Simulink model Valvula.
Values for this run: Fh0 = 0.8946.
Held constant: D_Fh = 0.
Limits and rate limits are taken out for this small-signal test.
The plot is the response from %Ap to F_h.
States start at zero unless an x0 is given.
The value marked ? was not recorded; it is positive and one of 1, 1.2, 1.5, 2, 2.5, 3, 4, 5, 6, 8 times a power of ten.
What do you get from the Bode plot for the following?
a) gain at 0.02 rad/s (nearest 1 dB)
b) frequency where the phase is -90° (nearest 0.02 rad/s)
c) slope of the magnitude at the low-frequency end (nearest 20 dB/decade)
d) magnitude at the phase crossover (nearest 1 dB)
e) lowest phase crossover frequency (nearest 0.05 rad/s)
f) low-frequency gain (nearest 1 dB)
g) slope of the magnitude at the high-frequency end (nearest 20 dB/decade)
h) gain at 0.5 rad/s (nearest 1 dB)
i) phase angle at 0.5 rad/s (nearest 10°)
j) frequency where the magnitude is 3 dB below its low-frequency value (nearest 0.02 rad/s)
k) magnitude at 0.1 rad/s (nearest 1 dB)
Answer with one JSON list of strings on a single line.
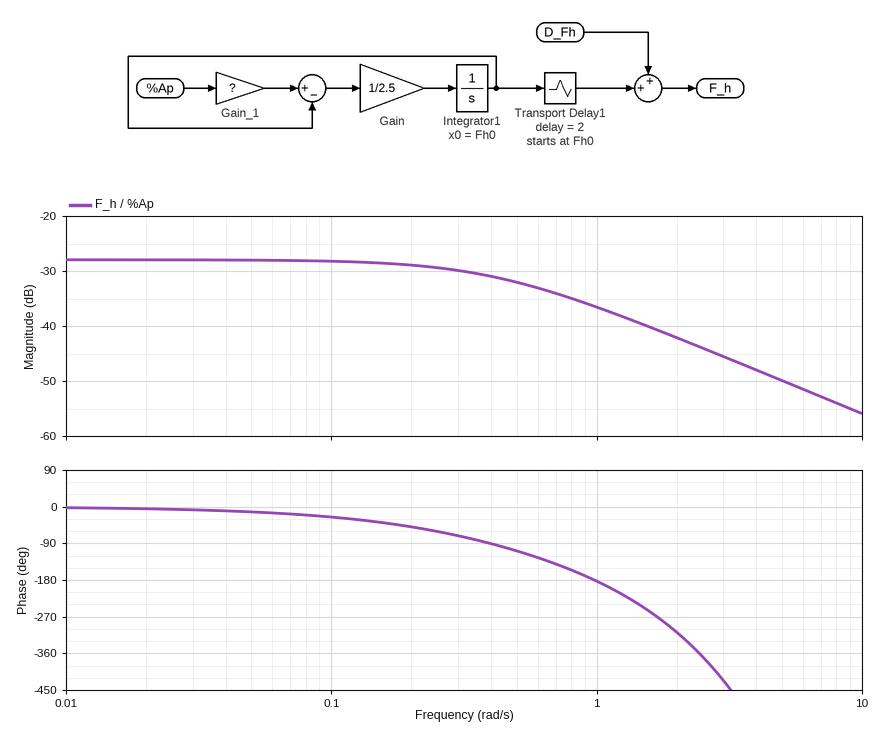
["-28 dB", "0.40 rad/s", "0 dB/decade", "-36 dB", "1.00 rad/s", "-28 dB", "-20 dB/decade", "-32 dB", "-110°", "0.40 rad/s", "-28 dB"]
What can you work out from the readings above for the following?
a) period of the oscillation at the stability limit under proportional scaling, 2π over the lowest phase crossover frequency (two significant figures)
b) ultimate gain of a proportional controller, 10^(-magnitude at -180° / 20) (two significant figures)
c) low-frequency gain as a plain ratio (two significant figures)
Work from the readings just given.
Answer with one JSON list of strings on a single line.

["6.3 s", "63", "0.040"]
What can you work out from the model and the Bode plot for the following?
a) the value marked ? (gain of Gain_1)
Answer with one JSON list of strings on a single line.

["0.04"]
